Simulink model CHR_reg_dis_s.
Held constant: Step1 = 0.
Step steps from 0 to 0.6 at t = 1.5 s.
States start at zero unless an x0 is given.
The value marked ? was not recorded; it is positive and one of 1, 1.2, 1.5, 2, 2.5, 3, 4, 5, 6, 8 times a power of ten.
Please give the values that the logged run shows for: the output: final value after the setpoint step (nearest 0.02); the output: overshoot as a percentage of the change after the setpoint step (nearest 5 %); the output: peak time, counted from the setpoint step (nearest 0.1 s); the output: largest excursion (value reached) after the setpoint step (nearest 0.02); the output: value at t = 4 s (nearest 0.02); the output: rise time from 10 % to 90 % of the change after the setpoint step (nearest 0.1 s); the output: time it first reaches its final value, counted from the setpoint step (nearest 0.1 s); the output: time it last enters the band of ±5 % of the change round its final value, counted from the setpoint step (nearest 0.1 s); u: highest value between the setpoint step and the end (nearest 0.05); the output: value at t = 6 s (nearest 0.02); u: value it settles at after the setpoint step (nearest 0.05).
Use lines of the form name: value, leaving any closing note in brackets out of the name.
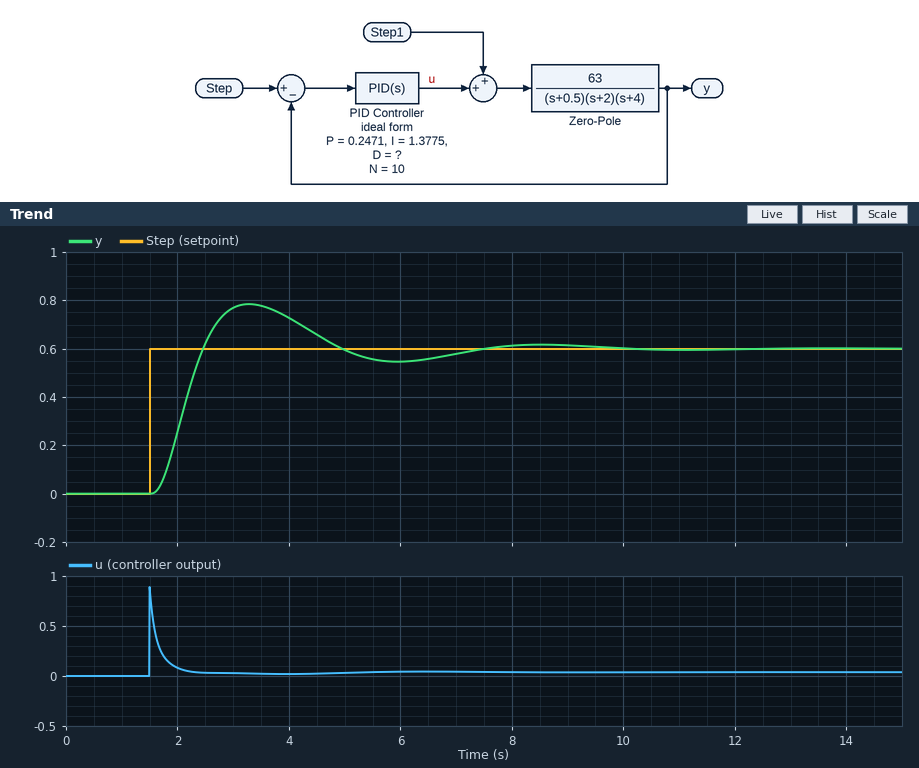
the output: final value after the setpoint step: 0.60
the output: overshoot as a percentage of the change after the setpoint step: 30 %
the output: peak time, counted from the setpoint step: 1.8 s
the output: largest excursion (value reached) after the setpoint step: 0.78
the output: value at t = 4 s: 0.72
the output: rise time from 10 % to 90 % of the change after the setpoint step: 0.6 s
the output: time it first reaches its final value, counted from the setpoint step: 1.0 s
the output: time it last enters the band of ±5 % of the change round its final value, counted from the setpoint step: 5.3 s
u: highest value between the setpoint step and the end: 0.90
the output: value at t = 6 s: 0.54
u: value it settles at after the setpoint step: 0.05
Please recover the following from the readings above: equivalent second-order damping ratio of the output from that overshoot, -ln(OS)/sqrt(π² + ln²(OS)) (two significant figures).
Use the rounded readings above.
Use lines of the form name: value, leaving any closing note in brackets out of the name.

equivalent second-order damping ratio of the output from that overshoot, -ln(OS)/sqrt(π² + ln²(OS)): 0.36
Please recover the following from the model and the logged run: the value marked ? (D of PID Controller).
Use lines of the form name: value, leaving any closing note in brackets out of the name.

the value marked ?: 0.5
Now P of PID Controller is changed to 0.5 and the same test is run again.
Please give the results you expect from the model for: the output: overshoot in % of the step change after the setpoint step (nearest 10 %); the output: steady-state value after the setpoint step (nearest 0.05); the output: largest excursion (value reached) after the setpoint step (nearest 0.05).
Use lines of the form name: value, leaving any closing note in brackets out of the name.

the output: overshoot in % of the step change after the setpoint step: 40 %
the output: steady-state value after the setpoint step: 0.60
the output: largest excursion (value reached) after the setpoint step: 0.85
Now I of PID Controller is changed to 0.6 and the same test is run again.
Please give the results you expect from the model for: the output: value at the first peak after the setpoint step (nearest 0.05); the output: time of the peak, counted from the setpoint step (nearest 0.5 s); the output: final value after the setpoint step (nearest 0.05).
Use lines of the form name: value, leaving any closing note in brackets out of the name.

the output: value at the first peak after the setpoint step: 0.65
the output: time of the peak, counted from the setpoint step: 3.0 s
the output: final value after the setpoint step: 0.60
